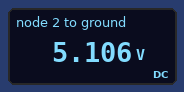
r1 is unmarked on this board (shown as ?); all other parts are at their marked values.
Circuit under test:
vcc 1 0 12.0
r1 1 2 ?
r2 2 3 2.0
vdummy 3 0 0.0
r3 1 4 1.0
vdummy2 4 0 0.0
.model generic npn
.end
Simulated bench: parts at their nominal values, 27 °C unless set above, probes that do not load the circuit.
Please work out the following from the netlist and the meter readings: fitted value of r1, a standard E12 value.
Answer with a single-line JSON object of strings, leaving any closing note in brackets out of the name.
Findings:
{"fitted value of r1, a standard E12 value": "2.7 Ω"}
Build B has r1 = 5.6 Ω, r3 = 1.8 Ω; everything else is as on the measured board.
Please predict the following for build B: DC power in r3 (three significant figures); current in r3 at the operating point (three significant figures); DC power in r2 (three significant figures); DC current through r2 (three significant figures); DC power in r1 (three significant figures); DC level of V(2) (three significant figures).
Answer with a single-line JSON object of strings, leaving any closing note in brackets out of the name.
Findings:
{"DC power in r3": "80.0 W", "current in r3 at the operating point": "6.67 A", "DC power in r2": "4.99 W", "DC current through r2": "1.58 A", "DC power in r1": "14.0 W", "DC level of V(2)": "3.16 V"}
